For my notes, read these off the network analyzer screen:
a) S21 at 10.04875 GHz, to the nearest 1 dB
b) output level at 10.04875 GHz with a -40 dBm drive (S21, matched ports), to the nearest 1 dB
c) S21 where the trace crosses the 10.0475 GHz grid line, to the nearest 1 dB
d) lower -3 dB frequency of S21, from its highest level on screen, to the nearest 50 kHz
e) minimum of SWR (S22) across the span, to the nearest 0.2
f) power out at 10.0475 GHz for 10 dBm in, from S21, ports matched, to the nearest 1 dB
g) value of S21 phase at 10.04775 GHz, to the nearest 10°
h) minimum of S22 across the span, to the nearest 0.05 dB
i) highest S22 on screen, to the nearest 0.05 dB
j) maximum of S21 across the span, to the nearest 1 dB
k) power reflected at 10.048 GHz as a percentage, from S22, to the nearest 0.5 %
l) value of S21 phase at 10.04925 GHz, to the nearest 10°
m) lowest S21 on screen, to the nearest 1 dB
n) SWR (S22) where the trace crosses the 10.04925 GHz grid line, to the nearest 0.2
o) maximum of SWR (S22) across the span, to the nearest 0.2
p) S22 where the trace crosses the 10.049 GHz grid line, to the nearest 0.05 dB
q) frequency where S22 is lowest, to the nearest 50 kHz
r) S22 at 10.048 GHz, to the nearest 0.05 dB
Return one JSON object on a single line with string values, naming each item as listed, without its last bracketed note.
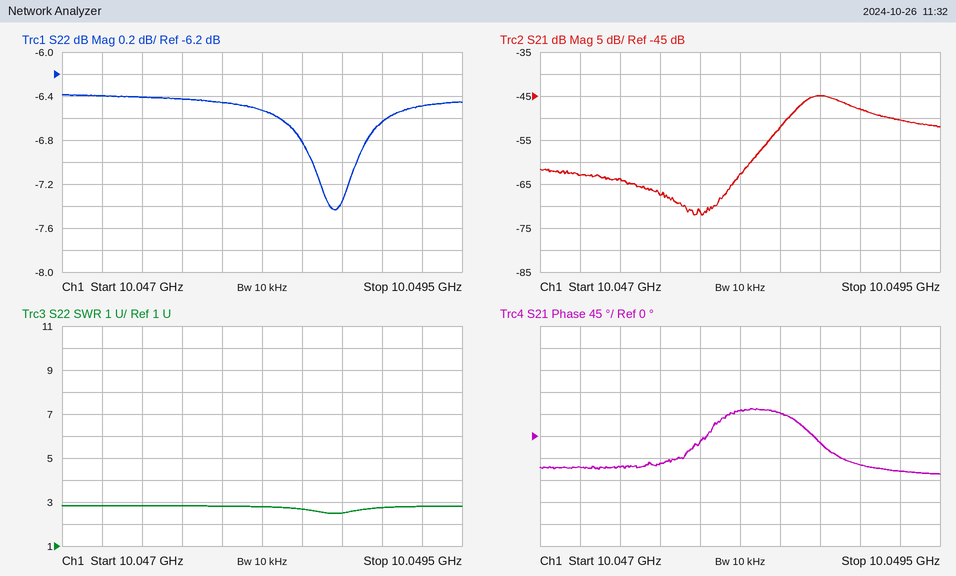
{"S21 at 10.04875 GHz, to the nearest 1 dB": "-45 dB", "output level at 10.04875 GHz with a -40 dBm drive (S21, matched ports), to the nearest 1 dB": "-85 dBm", "S21 where the trace crosses the 10.0475 GHz grid line, to the nearest 1 dB": "-64 dB", "lower -3 dB frequency of S21, from its highest level on screen, to the nearest 50 kHz": "10.04860 GHz", "minimum of SWR (S22) across the span, to the nearest 0.2": "2.4", "power out at 10.0475 GHz for 10 dBm in, from S21, ports matched, to the nearest 1 dB": "-54 dBm", "value of S21 phase at 10.04775 GHz, to the nearest 10°": "-60°", "minimum of S22 across the span, to the nearest 0.05 dB": "-7.45 dB", "highest S22 on screen, to the nearest 0.05 dB": "-6.40 dB", "maximum of S21 across the span, to the nearest 1 dB": "-45 dB", "power reflected at 10.048 GHz as a percentage, from S22, to the nearest 0.5 %": "22.5 %", "value of S21 phase at 10.04925 GHz, to the nearest 10°": "-70°", "lowest S21 on screen, to the nearest 1 dB": "-72 dB", "SWR (S22) where the trace crosses the 10.04925 GHz grid line, to the nearest 0.2": "2.8", "maximum of SWR (S22) across the span, to the nearest 0.2": "2.8", "S22 where the trace crosses the 10.049 GHz grid line, to the nearest 0.05 dB": "-6.65 dB", "frequency where S22 is lowest, to the nearest 50 kHz": "10.04870 GHz", "S22 at 10.048 GHz, to the nearest 0.05 dB": "-6.45 dB"}
